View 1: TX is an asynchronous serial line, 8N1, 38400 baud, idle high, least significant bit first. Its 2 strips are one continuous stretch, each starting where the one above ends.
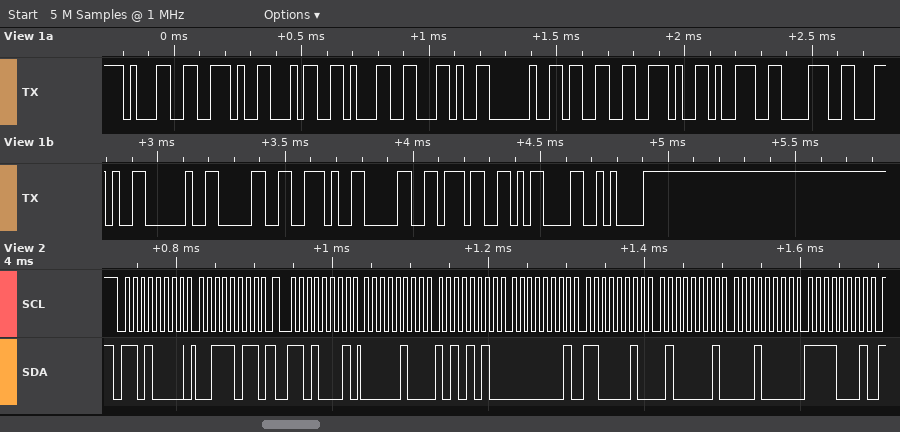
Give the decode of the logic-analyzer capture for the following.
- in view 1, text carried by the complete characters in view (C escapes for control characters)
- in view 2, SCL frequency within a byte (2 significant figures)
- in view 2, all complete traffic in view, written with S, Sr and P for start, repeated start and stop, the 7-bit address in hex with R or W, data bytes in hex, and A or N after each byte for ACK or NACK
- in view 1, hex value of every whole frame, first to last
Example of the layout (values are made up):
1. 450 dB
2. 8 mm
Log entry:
1. "1.41, 3.98, 0.07\r\n"
2. 100 kHz
3. S 68W A 3B A Sr 68R A 04 A AA A 01 A C2 A 41 A 10 A F1 A
4. 0x31 0x2E 0x34 0x31 0x2C 0x20 0x33 0x2E 0x39 0x38 0x2C 0x20 0x30 0x2E 0x30 0x37 0x0D 0x0A
